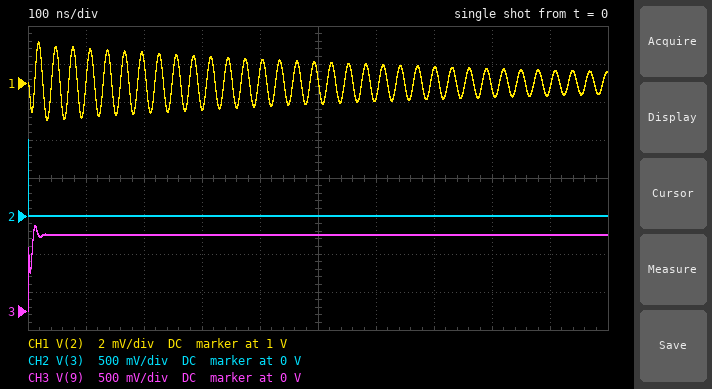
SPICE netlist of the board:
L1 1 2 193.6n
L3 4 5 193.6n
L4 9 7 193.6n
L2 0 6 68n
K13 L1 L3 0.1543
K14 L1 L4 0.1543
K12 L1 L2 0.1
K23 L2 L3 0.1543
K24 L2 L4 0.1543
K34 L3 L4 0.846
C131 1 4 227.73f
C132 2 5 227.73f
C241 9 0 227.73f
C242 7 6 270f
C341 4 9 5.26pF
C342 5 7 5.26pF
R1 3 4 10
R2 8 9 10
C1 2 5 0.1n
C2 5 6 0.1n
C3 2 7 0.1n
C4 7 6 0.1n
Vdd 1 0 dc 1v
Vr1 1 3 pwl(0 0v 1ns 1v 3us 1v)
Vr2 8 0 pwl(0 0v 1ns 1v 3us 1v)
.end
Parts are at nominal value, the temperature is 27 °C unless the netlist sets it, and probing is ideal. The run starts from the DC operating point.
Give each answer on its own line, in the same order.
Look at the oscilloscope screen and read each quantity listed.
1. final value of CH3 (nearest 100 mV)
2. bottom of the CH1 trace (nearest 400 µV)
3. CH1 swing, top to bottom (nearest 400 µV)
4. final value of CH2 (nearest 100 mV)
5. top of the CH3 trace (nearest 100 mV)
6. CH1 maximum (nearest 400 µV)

1.0 V
998.0 mV
4.0 mV
0 V
1.1 V
1.0020 V
